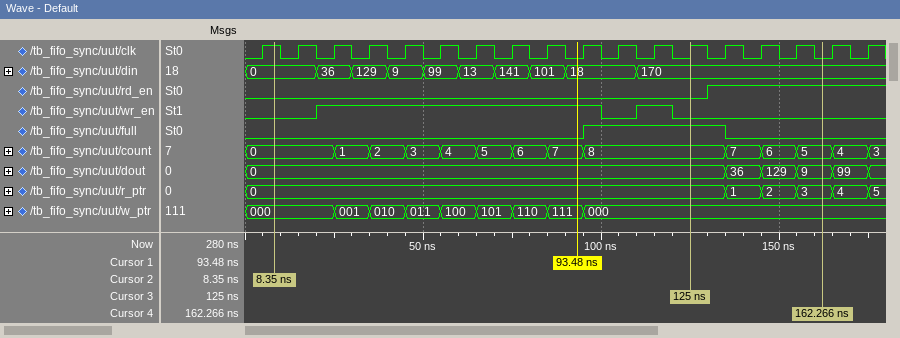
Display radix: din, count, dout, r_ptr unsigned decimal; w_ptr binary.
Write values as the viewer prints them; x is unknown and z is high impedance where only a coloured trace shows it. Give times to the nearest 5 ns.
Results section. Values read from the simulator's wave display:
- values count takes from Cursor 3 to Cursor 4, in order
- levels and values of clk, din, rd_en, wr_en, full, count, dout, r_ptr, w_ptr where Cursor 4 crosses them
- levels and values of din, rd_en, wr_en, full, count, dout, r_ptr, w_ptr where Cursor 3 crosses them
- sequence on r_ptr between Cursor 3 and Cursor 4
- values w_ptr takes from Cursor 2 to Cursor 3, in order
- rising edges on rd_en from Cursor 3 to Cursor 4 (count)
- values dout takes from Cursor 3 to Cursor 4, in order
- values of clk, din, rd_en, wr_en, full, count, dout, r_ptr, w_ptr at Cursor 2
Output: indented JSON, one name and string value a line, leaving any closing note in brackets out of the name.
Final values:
{
  "values count takes from Cursor 3 to Cursor 4, in order": "8, 7, 6, 5",
  "levels and values of clk, din, rd_en, wr_en, full, count, dout, r_ptr, w_ptr where Cursor 4 crosses them": "clk=0, din=170, rd_en=1, wr_en=0, full=0, count=5, dout=9, r_ptr=3, w_ptr=000",
  "levels and values of din, rd_en, wr_en, full, count, dout, r_ptr, w_ptr where Cursor 3 crosses them": "din=170, rd_en=0, wr_en=0, full=1, count=8, dout=0, r_ptr=0, w_ptr=000",
  "sequence on r_ptr between Cursor 3 and Cursor 4": "0, 1, 2, 3",
  "values w_ptr takes from Cursor 2 to Cursor 3, in order": "000, 001, 010, 011, 100, 101, 110, 111, 000",
  "rising edges on rd_en from Cursor 3 to Cursor 4": "1",
  "values dout takes from Cursor 3 to Cursor 4, in order": "0, 36, 129, 9",
  "values of clk, din, rd_en, wr_en, full, count, dout, r_ptr, w_ptr at Cursor 2": "clk=1, din=0, rd_en=0, wr_en=0, full=0, count=0, dout=0, r_ptr=0, w_ptr=000"
}
